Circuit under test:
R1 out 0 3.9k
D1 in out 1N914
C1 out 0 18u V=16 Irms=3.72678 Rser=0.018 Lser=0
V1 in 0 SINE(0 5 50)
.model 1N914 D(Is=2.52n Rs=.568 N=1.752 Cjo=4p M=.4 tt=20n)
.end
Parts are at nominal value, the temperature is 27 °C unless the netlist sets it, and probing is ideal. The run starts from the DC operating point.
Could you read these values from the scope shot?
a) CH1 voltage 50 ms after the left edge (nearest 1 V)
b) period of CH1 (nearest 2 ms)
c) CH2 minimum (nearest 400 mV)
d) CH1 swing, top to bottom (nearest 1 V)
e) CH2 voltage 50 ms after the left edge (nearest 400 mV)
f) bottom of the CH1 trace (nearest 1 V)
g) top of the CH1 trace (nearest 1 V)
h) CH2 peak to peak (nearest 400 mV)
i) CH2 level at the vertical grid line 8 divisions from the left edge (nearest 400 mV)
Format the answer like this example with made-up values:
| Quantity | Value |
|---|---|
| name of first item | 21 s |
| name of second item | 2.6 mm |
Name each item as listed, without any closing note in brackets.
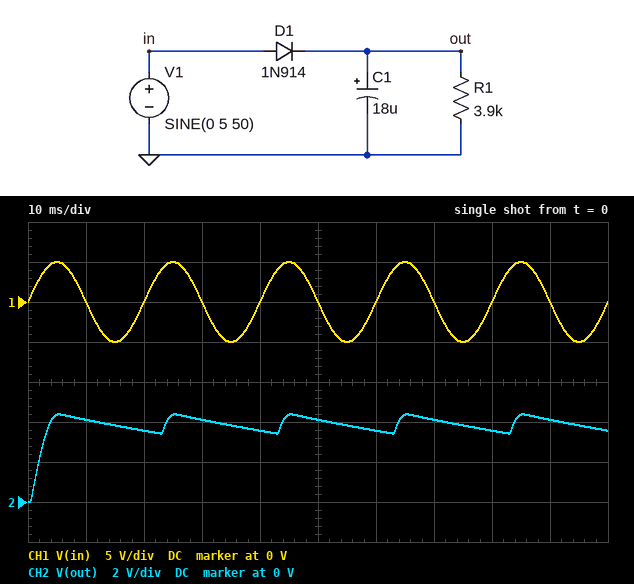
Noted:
| Quantity | Value |
|---|---|
| CH1 voltage 50 ms after the left edge | 0 V |
| period of CH1 | 20 ms |
| CH2 minimum | 0 V |
| CH1 swing, top to bottom | 10 V |
| CH2 voltage 50 ms after the left edge | 4.0 V |
| bottom of the CH1 trace | -5 V |
| top of the CH1 trace | 5 V |
| CH2 peak to peak | 4.4 V |
| CH2 level at the vertical grid line 8 divisions from the left edge | 3.6 V |
